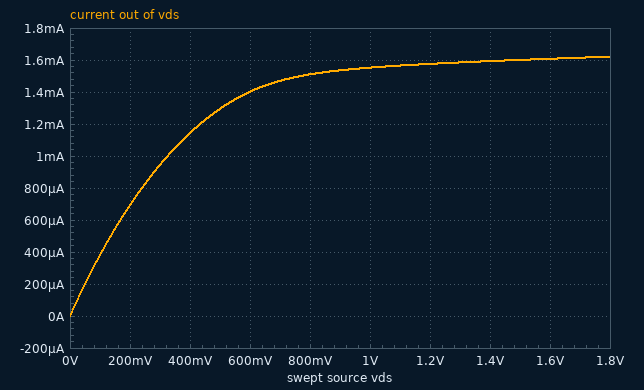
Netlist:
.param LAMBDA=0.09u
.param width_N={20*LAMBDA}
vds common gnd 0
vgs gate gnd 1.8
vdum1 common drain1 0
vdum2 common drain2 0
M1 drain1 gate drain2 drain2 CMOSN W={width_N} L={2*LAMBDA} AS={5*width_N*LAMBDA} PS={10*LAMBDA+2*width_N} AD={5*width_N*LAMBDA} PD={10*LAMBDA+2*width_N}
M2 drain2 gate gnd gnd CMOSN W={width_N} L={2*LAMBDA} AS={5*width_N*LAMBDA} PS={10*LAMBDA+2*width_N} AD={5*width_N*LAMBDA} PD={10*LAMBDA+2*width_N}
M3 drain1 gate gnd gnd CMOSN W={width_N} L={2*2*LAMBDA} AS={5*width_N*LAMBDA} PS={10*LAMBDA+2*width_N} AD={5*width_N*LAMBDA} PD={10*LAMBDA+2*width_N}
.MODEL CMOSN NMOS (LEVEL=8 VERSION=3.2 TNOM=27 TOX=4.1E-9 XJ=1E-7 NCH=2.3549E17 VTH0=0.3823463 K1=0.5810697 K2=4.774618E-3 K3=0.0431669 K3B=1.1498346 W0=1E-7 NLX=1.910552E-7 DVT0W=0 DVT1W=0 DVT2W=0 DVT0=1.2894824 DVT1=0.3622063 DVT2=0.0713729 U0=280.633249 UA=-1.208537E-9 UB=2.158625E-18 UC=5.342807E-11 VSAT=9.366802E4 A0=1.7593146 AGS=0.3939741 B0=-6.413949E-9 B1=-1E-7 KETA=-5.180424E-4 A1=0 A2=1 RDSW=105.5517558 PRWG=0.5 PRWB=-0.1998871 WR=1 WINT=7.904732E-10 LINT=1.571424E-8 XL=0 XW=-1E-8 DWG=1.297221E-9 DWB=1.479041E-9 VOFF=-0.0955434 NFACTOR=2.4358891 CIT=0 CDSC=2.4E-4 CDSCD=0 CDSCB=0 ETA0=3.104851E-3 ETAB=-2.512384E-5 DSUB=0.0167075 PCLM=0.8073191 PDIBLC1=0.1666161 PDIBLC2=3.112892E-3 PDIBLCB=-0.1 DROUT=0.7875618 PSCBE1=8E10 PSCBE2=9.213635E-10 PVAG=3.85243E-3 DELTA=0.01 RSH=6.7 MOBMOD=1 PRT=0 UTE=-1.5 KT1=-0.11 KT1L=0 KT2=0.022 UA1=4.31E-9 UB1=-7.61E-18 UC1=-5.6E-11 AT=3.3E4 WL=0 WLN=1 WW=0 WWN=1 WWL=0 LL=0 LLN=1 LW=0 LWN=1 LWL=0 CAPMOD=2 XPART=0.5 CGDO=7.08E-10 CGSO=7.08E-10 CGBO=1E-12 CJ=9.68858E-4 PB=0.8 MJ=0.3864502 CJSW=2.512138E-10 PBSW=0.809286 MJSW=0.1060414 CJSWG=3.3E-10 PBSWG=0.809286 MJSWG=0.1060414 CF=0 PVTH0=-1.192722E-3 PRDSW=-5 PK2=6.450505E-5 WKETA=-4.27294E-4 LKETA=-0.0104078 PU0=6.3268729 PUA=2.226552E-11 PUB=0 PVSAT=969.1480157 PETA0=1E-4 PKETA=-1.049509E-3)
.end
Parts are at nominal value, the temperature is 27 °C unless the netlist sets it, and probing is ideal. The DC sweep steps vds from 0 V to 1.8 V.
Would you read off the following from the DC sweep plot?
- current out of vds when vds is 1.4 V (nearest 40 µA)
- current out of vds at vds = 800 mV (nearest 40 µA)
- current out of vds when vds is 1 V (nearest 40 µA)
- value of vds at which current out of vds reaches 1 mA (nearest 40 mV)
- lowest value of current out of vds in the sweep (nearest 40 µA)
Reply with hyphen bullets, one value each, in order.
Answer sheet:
- 1.60 mA
- 1.52 mA
- 1.56 mA
- 320 mV
- 0 A
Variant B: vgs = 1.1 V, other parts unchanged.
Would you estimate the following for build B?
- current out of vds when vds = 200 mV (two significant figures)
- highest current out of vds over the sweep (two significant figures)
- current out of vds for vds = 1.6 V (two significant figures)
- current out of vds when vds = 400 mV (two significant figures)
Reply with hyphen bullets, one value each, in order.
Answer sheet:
- 360 µA
- 590 µA
- 580 µA
- 490 µA
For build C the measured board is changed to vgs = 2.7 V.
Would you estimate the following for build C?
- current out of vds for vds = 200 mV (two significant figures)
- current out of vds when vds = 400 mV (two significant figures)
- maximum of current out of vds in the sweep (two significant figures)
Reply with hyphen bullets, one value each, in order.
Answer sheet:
- 830 µA
- 1.5 mA
- 2.9 mA
